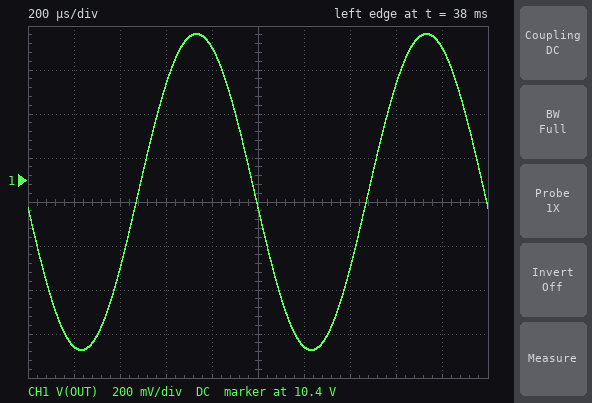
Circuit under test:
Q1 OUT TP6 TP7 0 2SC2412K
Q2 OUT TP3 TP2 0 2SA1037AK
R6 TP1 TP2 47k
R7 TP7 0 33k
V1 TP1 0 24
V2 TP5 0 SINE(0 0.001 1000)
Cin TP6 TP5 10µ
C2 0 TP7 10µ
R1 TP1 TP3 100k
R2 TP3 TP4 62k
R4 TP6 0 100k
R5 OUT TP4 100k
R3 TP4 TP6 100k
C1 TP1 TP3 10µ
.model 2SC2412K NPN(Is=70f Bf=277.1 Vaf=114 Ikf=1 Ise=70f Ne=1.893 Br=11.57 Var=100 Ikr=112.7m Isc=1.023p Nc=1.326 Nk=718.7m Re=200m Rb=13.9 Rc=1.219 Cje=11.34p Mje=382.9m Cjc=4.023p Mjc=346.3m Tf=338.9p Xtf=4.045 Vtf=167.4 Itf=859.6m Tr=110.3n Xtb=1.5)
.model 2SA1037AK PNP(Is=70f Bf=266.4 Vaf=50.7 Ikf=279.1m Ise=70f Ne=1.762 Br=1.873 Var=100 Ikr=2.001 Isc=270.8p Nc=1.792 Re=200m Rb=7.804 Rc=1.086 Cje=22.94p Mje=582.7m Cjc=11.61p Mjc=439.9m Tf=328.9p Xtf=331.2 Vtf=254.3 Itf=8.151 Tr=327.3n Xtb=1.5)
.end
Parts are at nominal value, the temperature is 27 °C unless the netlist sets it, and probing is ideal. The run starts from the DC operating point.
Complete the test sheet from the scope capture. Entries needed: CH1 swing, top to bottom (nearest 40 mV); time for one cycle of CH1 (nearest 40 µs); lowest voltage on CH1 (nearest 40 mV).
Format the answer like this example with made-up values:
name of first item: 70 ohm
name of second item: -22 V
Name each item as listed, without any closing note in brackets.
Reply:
CH1 swing, top to bottom: 1.44 V
time for one cycle of CH1: 1.00 ms
lowest voltage on CH1: 9.64 V
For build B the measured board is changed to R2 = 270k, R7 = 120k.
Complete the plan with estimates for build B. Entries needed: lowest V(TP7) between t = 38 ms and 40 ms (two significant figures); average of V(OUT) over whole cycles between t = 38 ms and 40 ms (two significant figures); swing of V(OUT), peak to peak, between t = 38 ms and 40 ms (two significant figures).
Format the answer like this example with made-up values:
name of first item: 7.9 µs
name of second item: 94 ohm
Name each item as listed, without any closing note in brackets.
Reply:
lowest V(TP7) between t = 38 ms and 40 ms: 5.0 V
average of V(OUT) over whole cycles between t = 38 ms and 40 ms: 13 V
swing of V(OUT), peak to peak, between t = 38 ms and 40 ms: 520 mV
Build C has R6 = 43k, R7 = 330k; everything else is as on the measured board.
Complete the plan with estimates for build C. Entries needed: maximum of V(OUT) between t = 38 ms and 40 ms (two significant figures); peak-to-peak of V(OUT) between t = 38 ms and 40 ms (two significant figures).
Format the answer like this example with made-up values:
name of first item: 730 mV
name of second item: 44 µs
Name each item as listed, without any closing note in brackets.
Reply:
maximum of V(OUT) between t = 38 ms and 40 ms: 21 V
peak-to-peak of V(OUT) between t = 38 ms and 40 ms: 5.2 mV
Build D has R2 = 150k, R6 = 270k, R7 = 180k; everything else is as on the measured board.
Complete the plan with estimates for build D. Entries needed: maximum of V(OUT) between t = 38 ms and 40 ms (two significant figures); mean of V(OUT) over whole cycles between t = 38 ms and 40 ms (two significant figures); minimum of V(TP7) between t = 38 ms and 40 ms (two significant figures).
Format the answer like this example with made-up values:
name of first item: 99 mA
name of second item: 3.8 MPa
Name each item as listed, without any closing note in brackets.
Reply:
maximum of V(OUT) between t = 38 ms and 40 ms: 9.5 V
mean of V(OUT) over whole cycles between t = 38 ms and 40 ms: 9.4 V
minimum of V(TP7) between t = 38 ms and 40 ms: 4.5 V
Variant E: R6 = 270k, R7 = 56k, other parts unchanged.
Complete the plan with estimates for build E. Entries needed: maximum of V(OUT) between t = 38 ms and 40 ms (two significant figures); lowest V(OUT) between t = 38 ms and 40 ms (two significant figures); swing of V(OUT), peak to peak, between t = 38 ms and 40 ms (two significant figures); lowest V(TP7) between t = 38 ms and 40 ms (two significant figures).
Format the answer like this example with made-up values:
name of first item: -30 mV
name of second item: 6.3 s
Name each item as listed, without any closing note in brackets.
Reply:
maximum of V(OUT) between t = 38 ms and 40 ms: 5.5 V
lowest V(OUT) between t = 38 ms and 40 ms: 4.8 V
swing of V(OUT), peak to peak, between t = 38 ms and 40 ms: 720 mV
lowest V(TP7) between t = 38 ms and 40 ms: 4.2 V
